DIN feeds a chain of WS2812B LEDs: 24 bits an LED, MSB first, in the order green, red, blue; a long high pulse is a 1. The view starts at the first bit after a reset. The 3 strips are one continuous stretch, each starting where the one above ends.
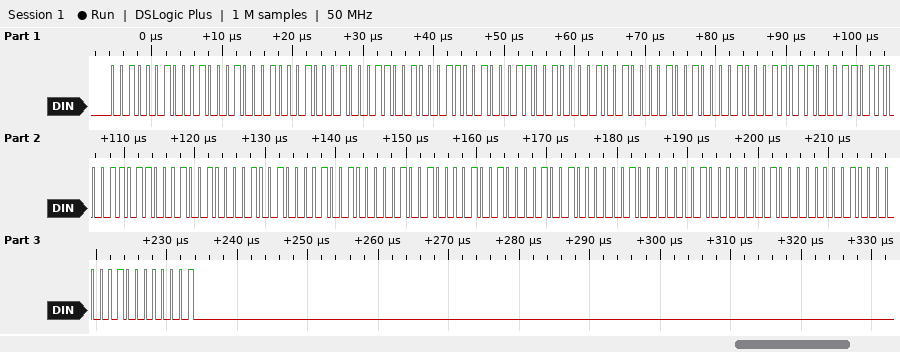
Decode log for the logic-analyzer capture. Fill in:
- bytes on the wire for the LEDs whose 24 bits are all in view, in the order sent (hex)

22 22 22 23 23 23 21 21 21 1B 1B 1B 12 12 12 09 09 09 02 02 02 01 01 01
